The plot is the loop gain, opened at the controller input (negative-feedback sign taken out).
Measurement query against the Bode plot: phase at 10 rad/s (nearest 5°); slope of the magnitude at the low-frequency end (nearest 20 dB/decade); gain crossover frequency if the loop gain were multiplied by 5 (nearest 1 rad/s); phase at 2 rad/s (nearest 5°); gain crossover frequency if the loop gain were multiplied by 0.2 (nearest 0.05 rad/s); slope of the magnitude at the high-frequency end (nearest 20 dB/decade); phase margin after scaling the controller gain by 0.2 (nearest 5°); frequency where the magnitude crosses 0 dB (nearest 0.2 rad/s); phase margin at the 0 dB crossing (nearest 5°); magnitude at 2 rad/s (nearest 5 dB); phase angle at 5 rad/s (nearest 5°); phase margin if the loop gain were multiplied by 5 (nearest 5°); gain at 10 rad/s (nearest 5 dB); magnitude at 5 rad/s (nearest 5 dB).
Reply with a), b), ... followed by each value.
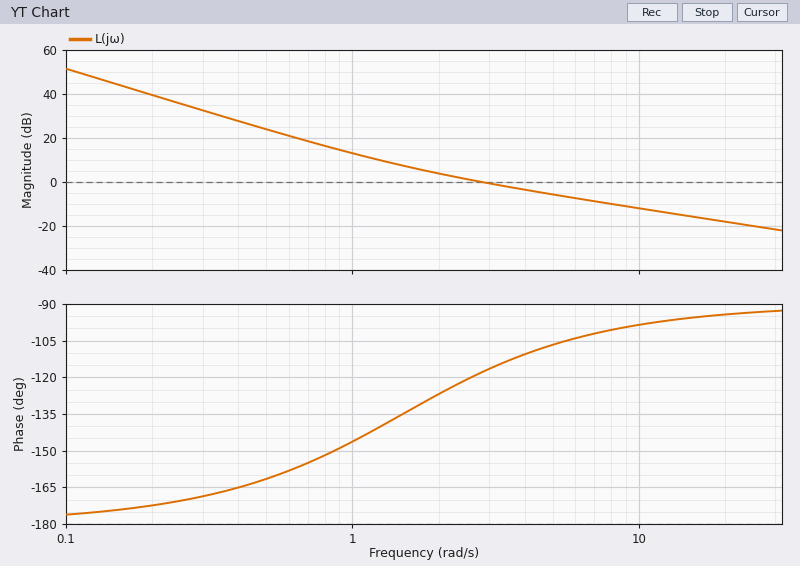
a) -100°
b) -40 dB/decade
c) 13 rad/s
d) -125°
e) 0.95 rad/s
f) -20 dB/decade
g) 30°
h) 2.8 rad/s
i) 60°
j) 5 dB
k) -105°
l) 85°
m) -10 dB
n) -5 dB
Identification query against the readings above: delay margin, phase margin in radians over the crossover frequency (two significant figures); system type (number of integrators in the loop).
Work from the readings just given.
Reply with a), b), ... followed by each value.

a) 0.37 s
b) 2
